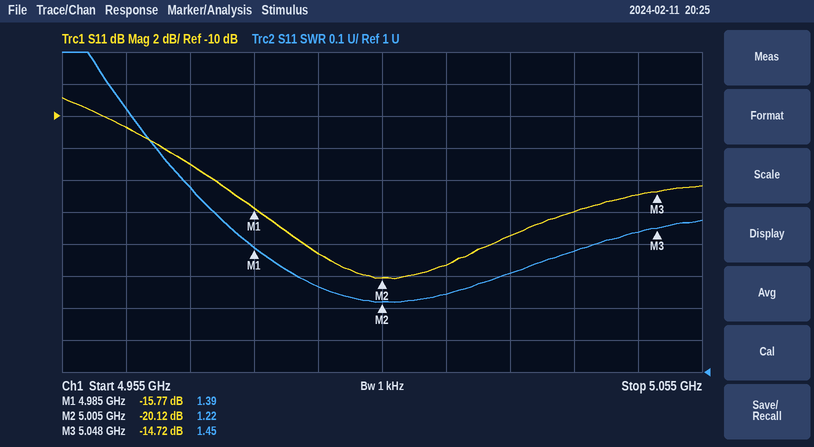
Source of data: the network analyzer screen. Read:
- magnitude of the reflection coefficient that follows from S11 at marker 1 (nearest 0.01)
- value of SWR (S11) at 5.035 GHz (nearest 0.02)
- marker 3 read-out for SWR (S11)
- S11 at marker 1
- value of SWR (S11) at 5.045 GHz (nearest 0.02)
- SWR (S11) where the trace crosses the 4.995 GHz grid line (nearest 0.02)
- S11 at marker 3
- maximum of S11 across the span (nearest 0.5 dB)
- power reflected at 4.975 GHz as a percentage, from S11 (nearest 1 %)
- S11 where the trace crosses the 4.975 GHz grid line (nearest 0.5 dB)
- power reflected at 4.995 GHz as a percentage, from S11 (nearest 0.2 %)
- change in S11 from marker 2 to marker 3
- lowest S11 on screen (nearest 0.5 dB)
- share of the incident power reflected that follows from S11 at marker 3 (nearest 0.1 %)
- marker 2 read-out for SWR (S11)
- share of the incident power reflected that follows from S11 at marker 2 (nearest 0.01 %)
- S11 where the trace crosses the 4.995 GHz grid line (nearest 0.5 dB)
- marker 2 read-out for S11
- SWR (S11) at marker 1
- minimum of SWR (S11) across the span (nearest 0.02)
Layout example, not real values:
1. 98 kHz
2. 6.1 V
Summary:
1. 0.16
2. 1.38
3. 1.45
4. -15.77 dB
5. 1.44
6. 1.26
7. -14.72 dB
8. -9.0 dB
9. 5 %
10. -13.0 dB
11. 1.4 %
12. 5.40 dB
13. -20.0 dB
14. 3.4 %
15. 1.22
16. 0.97 %
17. -18.5 dB
18. -20.12 dB
19. 1.39
20. 1.22
